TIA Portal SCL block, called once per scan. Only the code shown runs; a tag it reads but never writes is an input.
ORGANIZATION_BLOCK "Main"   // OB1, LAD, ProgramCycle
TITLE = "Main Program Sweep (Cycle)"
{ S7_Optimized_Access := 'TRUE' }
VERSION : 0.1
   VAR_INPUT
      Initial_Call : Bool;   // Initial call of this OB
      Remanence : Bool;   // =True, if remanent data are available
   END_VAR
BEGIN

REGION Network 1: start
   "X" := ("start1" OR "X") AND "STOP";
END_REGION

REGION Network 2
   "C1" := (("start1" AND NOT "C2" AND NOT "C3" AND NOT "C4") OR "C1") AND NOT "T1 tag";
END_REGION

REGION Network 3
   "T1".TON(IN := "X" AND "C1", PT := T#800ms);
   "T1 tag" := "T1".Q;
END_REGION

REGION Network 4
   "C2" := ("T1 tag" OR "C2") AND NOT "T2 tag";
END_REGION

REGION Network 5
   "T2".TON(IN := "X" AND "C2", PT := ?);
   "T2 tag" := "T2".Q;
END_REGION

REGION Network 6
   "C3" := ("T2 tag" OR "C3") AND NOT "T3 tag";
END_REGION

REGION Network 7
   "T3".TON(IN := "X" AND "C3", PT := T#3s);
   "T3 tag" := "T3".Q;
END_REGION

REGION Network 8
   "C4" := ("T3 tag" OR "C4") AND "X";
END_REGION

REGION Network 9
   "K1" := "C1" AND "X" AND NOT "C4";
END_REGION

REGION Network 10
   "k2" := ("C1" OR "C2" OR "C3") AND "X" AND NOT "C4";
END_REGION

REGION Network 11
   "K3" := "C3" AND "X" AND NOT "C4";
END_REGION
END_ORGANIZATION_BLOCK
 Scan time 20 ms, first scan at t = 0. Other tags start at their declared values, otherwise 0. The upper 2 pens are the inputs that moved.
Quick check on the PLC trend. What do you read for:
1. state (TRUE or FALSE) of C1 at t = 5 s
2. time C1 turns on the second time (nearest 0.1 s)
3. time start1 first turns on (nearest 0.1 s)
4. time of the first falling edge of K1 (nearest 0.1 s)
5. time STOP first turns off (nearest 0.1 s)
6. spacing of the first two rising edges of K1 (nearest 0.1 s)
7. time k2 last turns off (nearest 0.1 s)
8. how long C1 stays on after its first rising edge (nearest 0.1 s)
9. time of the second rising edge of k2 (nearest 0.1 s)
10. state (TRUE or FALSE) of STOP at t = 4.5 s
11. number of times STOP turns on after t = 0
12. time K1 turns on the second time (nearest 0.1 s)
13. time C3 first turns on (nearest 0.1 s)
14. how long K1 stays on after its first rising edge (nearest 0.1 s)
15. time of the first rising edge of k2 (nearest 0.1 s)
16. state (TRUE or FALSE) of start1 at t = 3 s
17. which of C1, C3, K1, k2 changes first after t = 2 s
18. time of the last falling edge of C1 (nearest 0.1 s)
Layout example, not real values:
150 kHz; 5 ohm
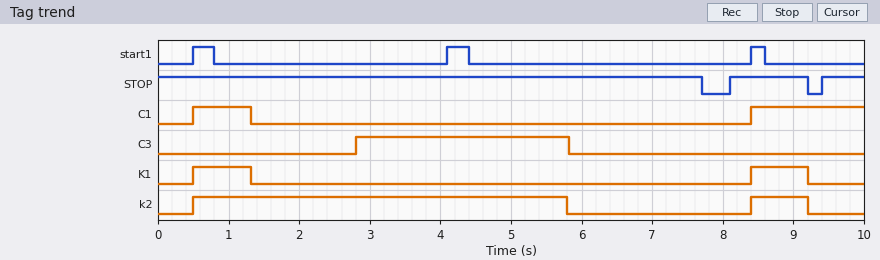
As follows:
FALSE; 8.4 s; 0.5 s; 1.3 s; 7.7 s; 7.9 s; 9.2 s; 0.8 s; 8.4 s; TRUE; 2; 8.4 s; 2.8 s; 0.8 s; 0.5 s; FALSE; C3; 1.3 s
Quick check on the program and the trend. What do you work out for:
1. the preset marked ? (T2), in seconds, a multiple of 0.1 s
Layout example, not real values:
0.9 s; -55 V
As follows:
1.5 s
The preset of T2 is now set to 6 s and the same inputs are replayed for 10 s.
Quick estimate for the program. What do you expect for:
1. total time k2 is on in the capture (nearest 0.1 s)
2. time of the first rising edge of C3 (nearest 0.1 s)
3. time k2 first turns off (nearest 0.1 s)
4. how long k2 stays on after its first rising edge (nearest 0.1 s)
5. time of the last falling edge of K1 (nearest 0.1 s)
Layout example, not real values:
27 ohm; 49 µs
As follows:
8.0 s; 7.3 s; 7.7 s; 7.2 s; 1.3 s
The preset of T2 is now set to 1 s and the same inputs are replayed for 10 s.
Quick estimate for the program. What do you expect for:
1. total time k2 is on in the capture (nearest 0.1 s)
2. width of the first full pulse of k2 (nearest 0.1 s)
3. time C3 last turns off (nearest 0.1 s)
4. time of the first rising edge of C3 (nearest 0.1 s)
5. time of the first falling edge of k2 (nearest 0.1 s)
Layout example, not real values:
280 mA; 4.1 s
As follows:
5.6 s; 4.8 s; 5.3 s; 2.3 s; 5.3 s
